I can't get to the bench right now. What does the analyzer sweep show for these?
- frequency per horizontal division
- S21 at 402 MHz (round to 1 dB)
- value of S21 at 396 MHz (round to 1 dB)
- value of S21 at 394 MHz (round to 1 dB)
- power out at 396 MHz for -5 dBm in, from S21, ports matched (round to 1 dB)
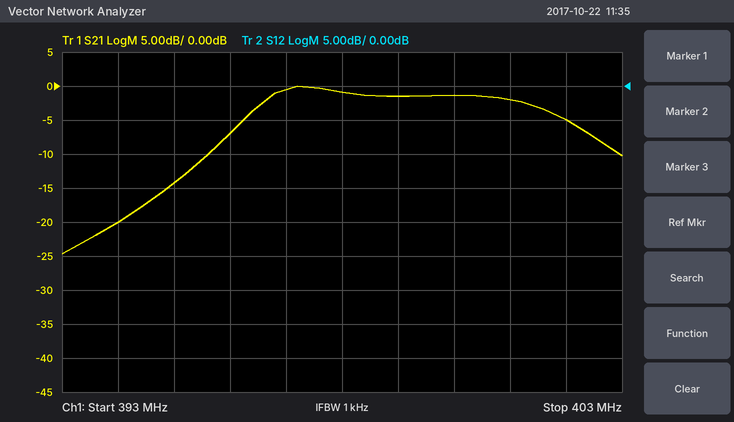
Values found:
1 MHz
-5 dB
-7 dB
-20 dB
-12 dBm
